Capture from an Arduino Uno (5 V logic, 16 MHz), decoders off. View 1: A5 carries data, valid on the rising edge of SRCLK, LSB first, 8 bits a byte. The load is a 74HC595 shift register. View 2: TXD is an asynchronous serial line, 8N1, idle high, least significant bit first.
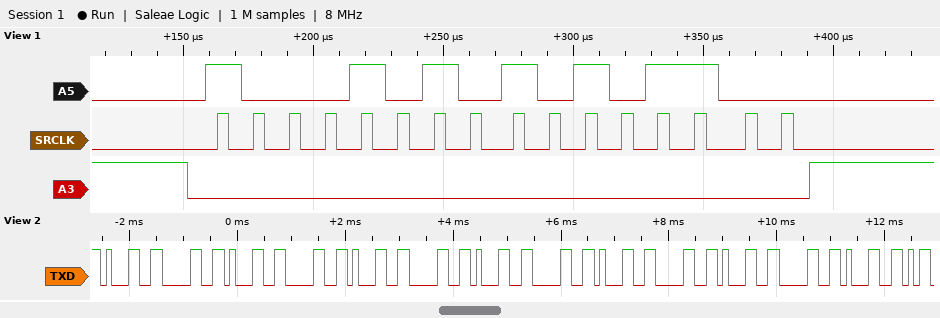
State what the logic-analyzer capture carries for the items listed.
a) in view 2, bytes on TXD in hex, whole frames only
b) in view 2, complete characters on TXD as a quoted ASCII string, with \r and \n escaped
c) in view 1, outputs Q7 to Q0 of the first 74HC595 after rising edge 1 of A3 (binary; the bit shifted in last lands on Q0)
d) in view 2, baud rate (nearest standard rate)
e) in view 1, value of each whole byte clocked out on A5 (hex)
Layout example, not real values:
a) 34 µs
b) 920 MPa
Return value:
a) 0x31 0x30 0x31 0x30 0x31 0x30 0x31 0x30 0x31 0x30 0x31 0x30 0x31
b) "1010101010101"
c) 10101100
d) 9600 baud
e) 0x51 0x35
